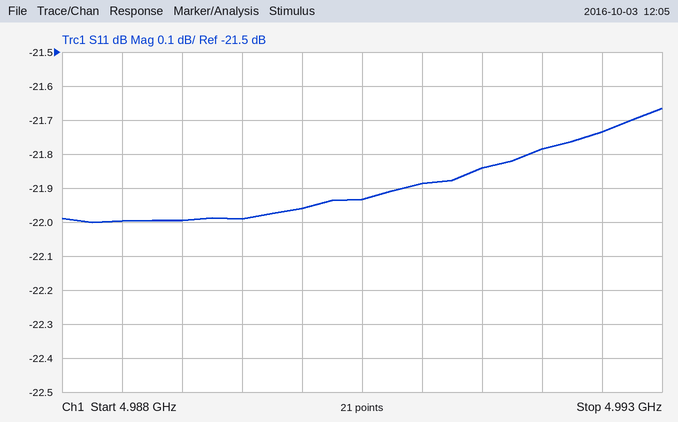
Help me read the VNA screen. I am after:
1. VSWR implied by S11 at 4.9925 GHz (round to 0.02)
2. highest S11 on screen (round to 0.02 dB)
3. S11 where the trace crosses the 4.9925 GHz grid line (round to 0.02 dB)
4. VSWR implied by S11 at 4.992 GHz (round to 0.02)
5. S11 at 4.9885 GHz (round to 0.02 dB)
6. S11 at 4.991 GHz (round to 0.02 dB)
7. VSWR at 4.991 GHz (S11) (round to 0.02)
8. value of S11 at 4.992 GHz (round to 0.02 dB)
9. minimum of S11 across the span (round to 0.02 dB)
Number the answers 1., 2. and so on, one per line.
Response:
1. 1.18
2. -21.66 dB
3. -21.74 dB
4. 1.18
5. -22.00 dB
6. -21.88 dB
7. 1.18
8. -21.78 dB
9. -22.00 dB
